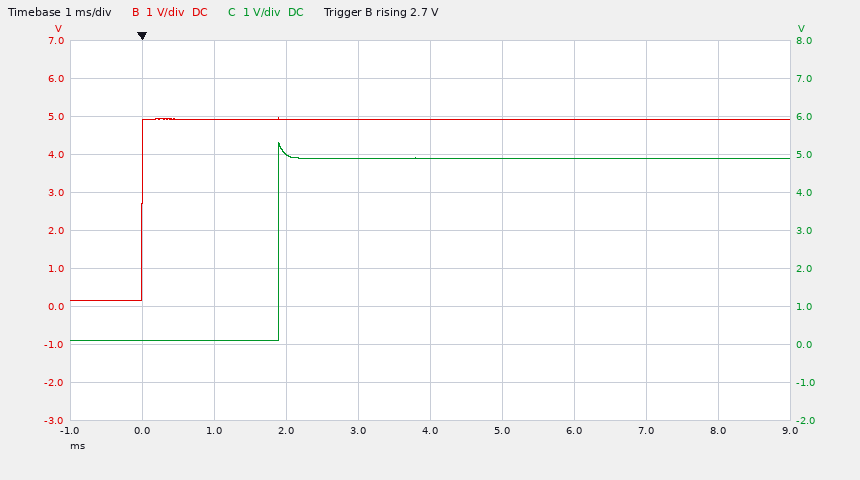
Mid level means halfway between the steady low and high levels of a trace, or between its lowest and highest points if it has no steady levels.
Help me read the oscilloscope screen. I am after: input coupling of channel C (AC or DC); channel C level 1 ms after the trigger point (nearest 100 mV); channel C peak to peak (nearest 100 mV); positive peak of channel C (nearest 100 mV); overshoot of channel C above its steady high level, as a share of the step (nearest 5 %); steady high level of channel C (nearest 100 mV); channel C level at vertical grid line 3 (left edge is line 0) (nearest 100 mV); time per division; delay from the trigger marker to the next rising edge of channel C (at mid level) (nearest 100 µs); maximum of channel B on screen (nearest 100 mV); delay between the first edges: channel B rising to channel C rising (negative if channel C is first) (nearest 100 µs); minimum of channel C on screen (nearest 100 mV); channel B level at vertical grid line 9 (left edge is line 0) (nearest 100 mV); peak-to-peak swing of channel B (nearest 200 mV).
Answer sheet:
DC
100 mV
5.2 V
5.3 V
10 %
4.9 V
5.0 V
1 ms
1.9 ms
5.0 V
+1.9 ms
100 mV
4.9 V
4.8 V
